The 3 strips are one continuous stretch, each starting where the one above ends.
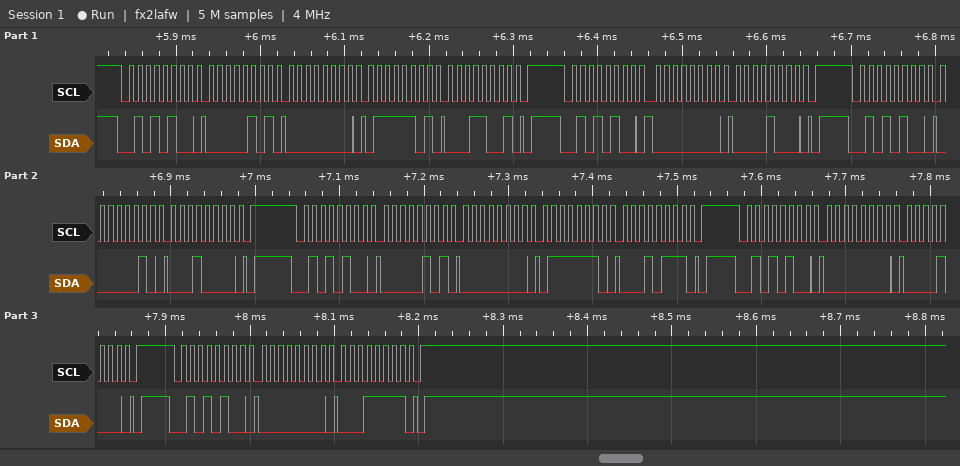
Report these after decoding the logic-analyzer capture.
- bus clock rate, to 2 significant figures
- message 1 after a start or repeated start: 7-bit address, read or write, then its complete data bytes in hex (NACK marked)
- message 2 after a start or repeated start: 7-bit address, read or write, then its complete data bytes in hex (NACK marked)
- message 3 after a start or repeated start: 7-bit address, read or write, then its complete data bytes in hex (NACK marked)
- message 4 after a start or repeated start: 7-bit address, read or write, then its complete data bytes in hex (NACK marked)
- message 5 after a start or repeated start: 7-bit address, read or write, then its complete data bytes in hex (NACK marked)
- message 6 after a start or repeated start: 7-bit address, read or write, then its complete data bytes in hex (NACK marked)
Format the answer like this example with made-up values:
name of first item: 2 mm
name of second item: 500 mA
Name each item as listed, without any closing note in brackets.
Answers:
bus clock rate, to 2 significant figures: 100 kHz
message 1 after a start or repeated start: 7-bit address, read or write, then its complete data bytes in hex: 0x2A write: 05 00 7D 19
message 2 after a start or repeated start: 7-bit address, read or write, then its complete data bytes in hex: 0x2A write: 00 08
message 3 after a start or repeated start: 7-bit address, read or write, then its complete data bytes in hex: 0x2A write: 02 10
message 4 after a start or repeated start: 7-bit address, read or write, then its complete data bytes in hex: 0x2A write: 05 00 7E 17
message 5 after a start or repeated start: 7-bit address, read or write, then its complete data bytes in hex: 0x2A write: 00 08
message 6 after a start or repeated start: 7-bit address, read or write, then its complete data bytes in hex: 0x2A write: 00 1F
